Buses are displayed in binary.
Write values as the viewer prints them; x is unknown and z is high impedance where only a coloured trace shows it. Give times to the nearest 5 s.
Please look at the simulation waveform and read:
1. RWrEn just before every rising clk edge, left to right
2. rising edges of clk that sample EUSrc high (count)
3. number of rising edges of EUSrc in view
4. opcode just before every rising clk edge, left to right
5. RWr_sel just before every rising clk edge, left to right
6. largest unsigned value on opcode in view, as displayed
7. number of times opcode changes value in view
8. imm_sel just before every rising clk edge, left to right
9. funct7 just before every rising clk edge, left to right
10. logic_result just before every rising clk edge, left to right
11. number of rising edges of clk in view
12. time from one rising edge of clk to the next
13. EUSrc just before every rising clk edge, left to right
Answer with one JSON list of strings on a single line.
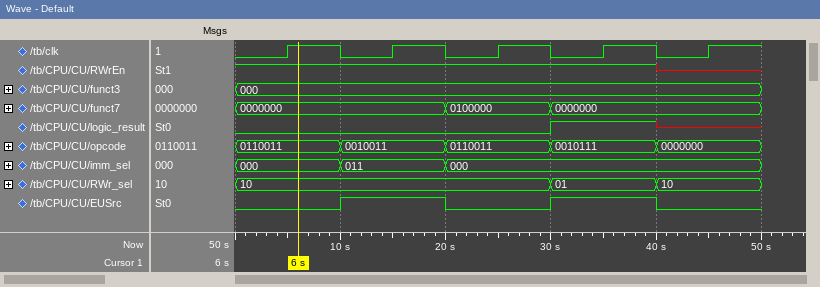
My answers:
["1 1 1 1 x", "2", "2", "0110011, 0010011, 0110011, 0010111, 0000000", "10, 10, 10, 01, 10", "0110011", "4", "000, 011, 000, 000, 000", "0000000, 0000000, 0100000, 0000000, 0000000", "0 0 0 1 x", "5", "10 s", "0 1 0 1 0"]
